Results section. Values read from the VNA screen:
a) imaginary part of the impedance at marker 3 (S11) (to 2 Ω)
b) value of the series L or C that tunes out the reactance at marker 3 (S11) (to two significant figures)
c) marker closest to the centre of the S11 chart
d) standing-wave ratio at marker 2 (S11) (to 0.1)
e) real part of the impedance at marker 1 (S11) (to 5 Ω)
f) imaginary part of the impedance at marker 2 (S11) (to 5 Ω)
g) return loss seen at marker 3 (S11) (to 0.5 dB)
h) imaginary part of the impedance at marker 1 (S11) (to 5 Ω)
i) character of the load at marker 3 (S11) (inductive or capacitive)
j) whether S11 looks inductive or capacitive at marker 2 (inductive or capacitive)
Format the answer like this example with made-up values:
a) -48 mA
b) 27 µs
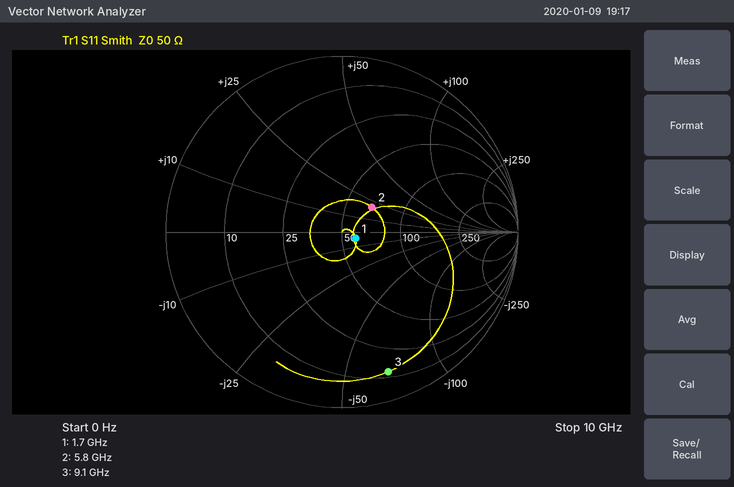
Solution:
a) -68 Ω
b) 1.2 nH
c) marker 1
d) 1.6
e) 60 Ω
f) +20 Ω
g) 1.5 dB
h) -5 Ω
i) capacitive
j) inductive
